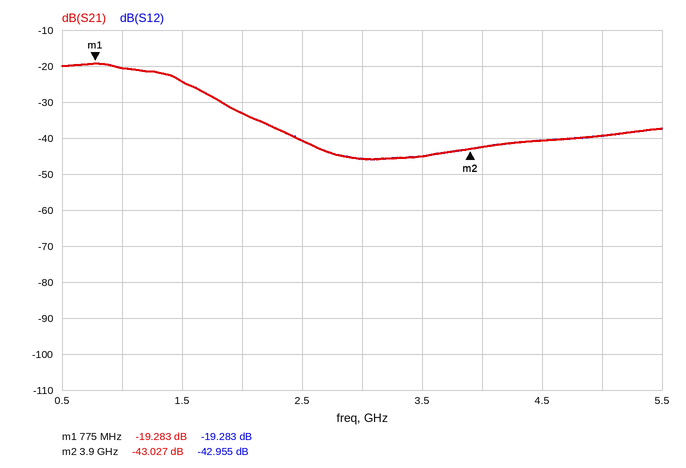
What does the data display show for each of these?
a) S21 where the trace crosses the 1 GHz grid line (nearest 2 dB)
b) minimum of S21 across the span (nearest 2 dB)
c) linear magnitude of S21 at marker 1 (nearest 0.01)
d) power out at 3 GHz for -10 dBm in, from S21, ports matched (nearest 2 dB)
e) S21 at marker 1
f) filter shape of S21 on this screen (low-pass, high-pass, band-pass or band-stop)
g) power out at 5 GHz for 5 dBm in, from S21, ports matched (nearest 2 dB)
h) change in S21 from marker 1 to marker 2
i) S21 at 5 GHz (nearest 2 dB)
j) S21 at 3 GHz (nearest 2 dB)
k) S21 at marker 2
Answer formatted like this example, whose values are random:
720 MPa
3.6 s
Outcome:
-20 dB
-46 dB
0.11
-56 dBm
-19.283 dB
low-pass
-34 dBm
-23.744 dB
-40 dB
-46 dB
-43.027 dB
